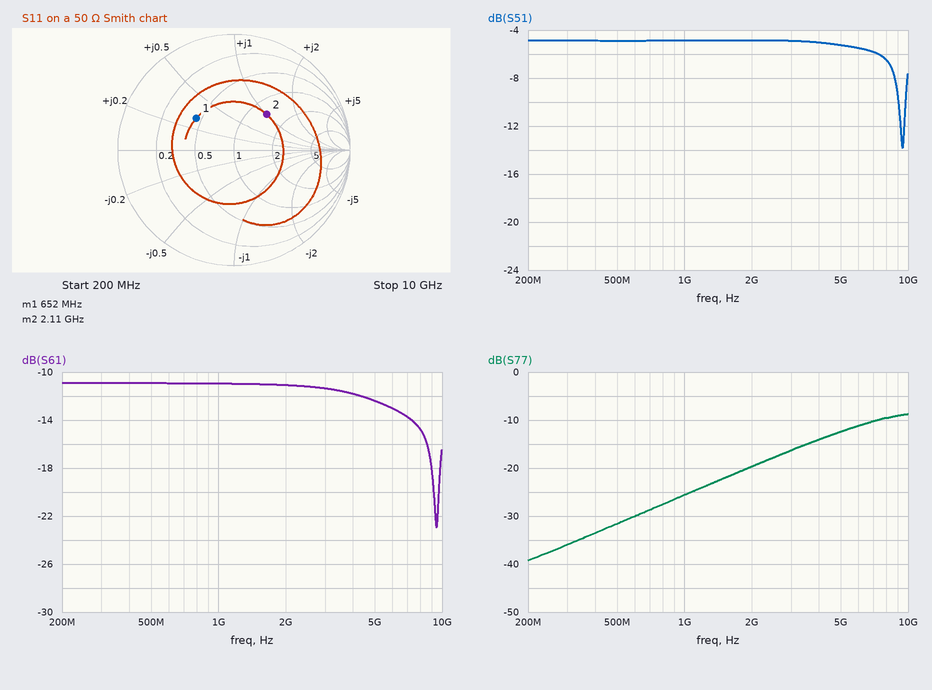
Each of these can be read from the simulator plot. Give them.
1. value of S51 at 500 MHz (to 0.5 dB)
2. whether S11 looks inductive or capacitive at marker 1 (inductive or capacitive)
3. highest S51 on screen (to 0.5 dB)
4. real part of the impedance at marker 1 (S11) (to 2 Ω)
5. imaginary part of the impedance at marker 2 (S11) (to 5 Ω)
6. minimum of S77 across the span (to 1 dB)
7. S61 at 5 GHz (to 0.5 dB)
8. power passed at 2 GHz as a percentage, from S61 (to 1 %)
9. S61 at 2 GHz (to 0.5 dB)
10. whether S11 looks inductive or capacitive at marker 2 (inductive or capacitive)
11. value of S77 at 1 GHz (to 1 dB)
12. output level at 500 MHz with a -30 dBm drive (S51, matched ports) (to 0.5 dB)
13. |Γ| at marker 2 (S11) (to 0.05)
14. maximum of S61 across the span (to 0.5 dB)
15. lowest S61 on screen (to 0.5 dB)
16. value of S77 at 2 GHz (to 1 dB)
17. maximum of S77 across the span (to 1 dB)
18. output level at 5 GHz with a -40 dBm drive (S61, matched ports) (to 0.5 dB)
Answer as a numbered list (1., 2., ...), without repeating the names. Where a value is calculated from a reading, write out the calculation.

1. -5.0 dB
2. inductive
3. -5.0 dB
4. 22 Ω
5. +50 Ω
6. -39 dB
7. -12.5 dB
8. 10^(-11/10) ≈ 8 %
9. -11.0 dB
10. inductive
11. -26 dB
12. -30 dBm + (-5.0 dB) = -35.0 dBm
13. 0.40
14. -11.0 dB
15. -23.0 dB
16. -20 dB
17. -9 dB
18. -40 dBm + (-12.5 dB) = -52.5 dBm
